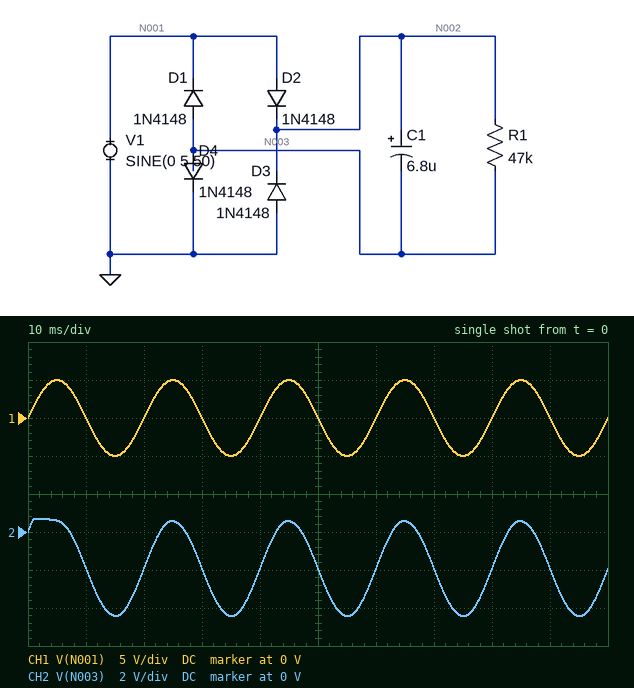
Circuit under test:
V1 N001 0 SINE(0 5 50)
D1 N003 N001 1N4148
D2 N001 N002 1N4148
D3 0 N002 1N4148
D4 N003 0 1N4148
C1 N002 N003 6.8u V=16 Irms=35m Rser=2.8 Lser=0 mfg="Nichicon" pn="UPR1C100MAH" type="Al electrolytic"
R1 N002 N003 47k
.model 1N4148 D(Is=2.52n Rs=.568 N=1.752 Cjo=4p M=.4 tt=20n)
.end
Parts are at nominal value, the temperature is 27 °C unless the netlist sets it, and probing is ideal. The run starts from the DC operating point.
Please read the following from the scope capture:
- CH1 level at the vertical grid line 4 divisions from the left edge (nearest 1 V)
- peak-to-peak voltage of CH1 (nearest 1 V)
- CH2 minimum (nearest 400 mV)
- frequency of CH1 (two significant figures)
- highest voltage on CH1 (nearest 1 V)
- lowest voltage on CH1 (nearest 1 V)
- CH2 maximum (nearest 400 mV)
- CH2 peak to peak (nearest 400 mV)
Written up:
0 V
10 V
-4.4 V
50 Hz
5 V
-5 V
800 mV
5.2 V
